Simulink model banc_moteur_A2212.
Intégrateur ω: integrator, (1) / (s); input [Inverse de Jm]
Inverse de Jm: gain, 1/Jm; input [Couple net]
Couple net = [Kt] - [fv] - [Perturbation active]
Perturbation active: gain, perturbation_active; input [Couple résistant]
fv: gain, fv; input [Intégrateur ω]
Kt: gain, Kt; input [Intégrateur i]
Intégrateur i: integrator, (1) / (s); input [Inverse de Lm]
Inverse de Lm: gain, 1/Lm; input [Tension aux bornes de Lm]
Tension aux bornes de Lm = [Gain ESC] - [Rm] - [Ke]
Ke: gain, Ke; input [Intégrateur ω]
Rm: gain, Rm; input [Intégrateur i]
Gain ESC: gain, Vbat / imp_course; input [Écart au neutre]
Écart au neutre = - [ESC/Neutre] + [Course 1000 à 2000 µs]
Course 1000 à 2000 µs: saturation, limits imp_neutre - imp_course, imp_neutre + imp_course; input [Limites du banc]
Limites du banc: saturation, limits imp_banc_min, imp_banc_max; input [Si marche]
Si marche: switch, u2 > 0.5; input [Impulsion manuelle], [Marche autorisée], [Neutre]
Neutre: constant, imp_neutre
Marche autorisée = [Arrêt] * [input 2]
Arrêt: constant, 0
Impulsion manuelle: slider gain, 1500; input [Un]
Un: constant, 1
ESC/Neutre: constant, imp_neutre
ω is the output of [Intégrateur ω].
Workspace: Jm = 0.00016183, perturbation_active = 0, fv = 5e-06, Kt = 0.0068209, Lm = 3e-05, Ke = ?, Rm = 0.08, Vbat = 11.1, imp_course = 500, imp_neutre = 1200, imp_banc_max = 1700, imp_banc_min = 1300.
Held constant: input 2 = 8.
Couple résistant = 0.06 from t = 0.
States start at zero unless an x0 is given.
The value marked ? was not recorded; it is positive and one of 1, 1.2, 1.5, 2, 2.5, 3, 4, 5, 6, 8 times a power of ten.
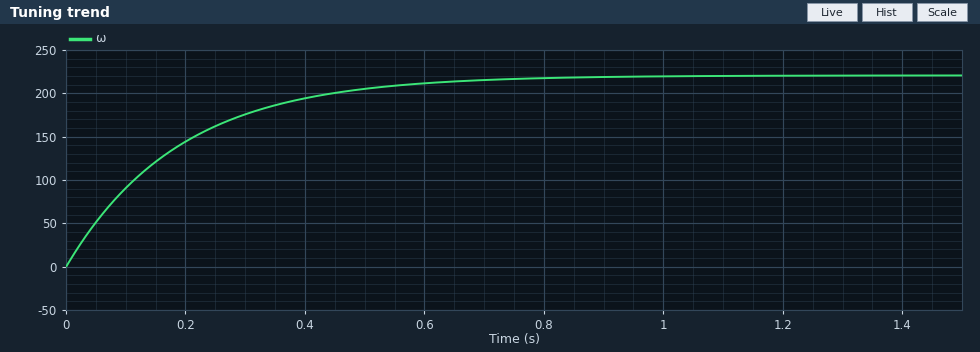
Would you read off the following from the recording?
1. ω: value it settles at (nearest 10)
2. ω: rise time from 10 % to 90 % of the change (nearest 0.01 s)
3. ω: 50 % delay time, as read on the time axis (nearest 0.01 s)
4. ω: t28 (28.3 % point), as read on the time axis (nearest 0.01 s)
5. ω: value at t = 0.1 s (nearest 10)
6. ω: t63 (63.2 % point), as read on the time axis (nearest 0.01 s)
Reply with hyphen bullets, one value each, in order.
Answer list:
- 220
- 0.41 s
- 0.13 s
- 0.06 s
- 90
- 0.19 s
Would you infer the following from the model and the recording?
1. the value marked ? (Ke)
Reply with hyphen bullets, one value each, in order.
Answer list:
- 0.01
